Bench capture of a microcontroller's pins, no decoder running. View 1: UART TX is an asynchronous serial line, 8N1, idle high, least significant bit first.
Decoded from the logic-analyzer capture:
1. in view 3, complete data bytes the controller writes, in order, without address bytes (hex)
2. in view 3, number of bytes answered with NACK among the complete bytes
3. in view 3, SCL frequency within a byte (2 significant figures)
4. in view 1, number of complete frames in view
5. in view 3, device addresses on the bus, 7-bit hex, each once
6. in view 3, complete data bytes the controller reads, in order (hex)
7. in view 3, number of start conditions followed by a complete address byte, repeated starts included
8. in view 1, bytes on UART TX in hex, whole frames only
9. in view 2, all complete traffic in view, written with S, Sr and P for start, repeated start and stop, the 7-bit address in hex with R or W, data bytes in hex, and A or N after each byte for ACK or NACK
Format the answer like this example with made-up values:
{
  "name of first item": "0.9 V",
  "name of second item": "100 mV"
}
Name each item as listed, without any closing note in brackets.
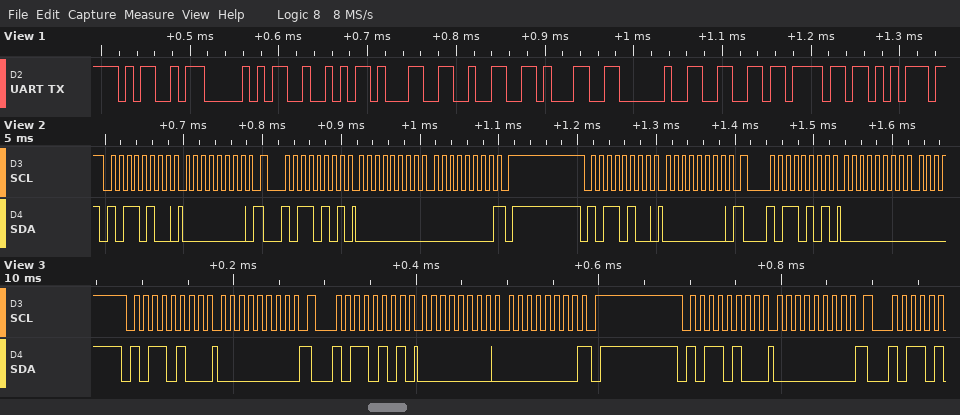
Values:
{
  "in view 3, complete data bytes the controller writes, in order, without address bytes": "00 00",
  "in view 3, number of bytes answered with NACK among the complete bytes": "1",
  "in view 3, SCL frequency within a byte": "100 kHz",
  "in view 1, number of complete frames in view": "10",
  "in view 3, device addresses on the bus, 7-bit hex, each once": "0x5A",
  "in view 3, complete data bytes the controller reads, in order": "00 00",
  "in view 3, number of start conditions followed by a complete address byte, repeated starts included": "3",
  "in view 1, bytes on UART TX in hex, whole frames only": "4D 50 52 31 32 31 20 66 6F 75",
  "in view 2, all complete traffic in view, written with S, Sr and P for start, repeated start and stop, the 7-bit address in hex with R or W, data bytes in hex, and A or N after each byte for ACK or NACK": "S 5AW A 00 A Sr 5AR A 00 A 00 N P S 5AW A 00 A Sr 5AR A 00 A"
}
